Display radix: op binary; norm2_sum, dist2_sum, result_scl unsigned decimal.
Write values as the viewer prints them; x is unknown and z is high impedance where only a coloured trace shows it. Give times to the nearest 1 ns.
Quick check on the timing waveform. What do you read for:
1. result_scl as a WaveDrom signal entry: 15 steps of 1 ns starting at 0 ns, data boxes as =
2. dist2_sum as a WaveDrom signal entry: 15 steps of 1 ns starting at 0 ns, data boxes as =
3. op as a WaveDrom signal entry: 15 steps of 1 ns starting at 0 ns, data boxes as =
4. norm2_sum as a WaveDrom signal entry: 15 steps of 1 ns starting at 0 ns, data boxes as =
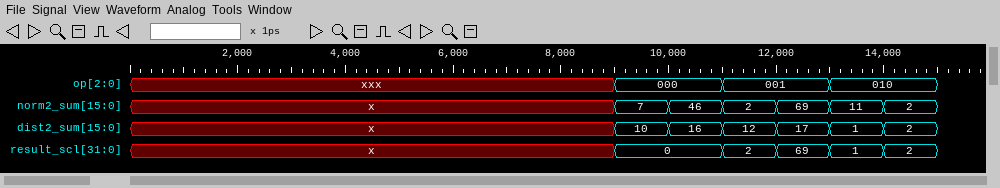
{name: 'result_scl', wave: 'x........=.====', data: '0 2 69 1 2'}
{name: 'dist2_sum', wave: 'x........======', data: '10 16 12 17 1 2'}
{name: 'op', wave: 'x........=.=.=.', data: '000 001 010'}
{name: 'norm2_sum', wave: 'x........======', data: '7 46 2 69 11 2'}
